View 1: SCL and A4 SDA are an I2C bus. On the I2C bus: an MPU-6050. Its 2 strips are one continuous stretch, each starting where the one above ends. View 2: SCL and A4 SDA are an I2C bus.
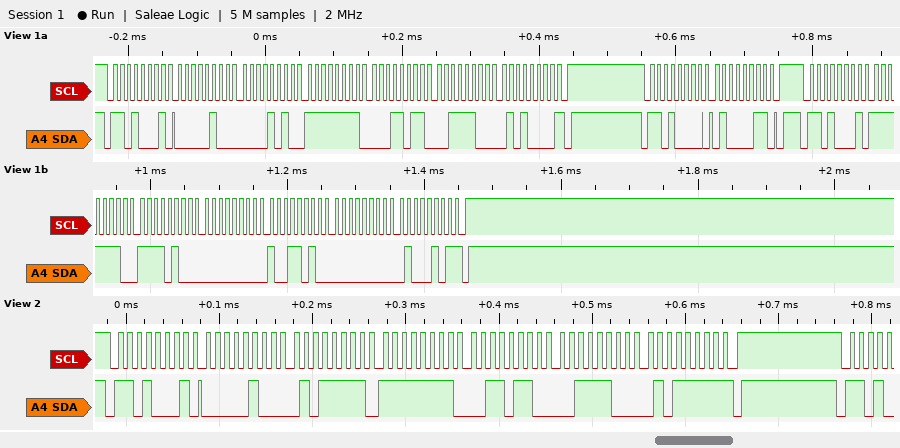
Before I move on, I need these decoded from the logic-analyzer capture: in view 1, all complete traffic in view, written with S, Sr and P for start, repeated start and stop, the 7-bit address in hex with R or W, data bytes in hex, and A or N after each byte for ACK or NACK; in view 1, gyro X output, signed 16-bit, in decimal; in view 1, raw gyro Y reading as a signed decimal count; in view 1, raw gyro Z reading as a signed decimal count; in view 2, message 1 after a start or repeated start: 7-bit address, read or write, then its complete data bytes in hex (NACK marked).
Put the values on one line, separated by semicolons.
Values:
S 68R A 04 A 0A A FF A 1B A 3C A 50 N P S 68W A 43 A P S 68R A FE A F4 A 00 A 9A A 00 A 45 N P; -268; 154; 69; 0x68 read: 04 5F FF 36 3C 5F NACK
